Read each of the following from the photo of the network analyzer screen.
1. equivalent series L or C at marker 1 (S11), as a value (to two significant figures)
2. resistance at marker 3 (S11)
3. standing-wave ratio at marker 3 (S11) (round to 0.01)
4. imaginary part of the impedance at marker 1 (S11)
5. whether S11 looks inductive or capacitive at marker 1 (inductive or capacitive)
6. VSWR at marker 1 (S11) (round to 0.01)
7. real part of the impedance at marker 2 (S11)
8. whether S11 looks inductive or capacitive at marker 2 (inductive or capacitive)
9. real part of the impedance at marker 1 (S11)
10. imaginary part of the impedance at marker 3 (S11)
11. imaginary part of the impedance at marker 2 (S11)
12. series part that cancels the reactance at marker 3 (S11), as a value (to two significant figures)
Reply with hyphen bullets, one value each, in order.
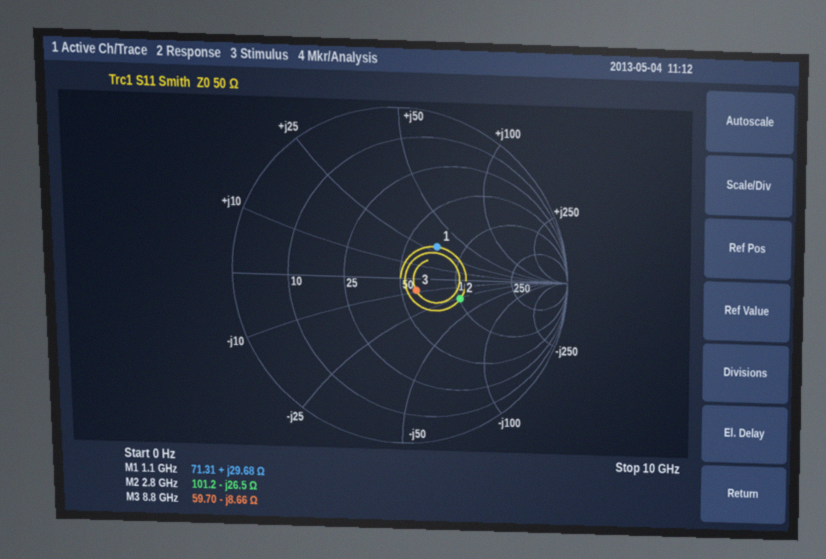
- 4.3 nH
- 59.70 Ω
- 1.27
- +29.68 Ω
- inductive
- 1.83
- 101.2 Ω
- capacitive
- 71.31 Ω
- -8.66 Ω
- -26.5 Ω
- 160 pH
